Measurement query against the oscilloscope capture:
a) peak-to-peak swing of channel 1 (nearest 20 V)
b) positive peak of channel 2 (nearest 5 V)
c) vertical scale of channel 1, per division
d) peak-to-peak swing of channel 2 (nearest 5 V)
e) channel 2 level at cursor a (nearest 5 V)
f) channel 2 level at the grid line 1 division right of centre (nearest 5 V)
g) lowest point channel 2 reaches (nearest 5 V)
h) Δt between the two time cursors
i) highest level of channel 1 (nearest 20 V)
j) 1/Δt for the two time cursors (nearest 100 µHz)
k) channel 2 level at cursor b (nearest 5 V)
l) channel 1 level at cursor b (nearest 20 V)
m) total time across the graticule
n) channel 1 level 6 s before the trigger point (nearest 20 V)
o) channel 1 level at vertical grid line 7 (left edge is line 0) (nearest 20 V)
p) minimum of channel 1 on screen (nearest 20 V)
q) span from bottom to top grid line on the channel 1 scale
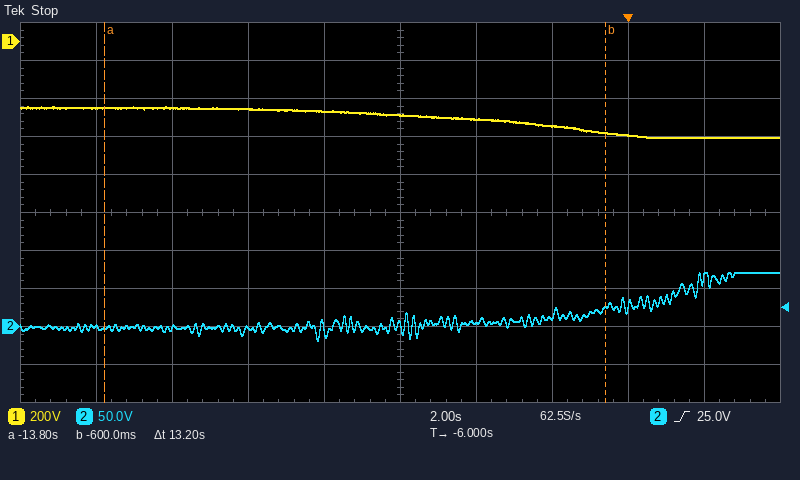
160 V
70 V
200 V
90 V
0 V
5 V
-20 V
13.2 s
-340 V
75.8 mHz
25 V
-480 V
20 s
-380 V
-440 V
-500 V
2 kV
